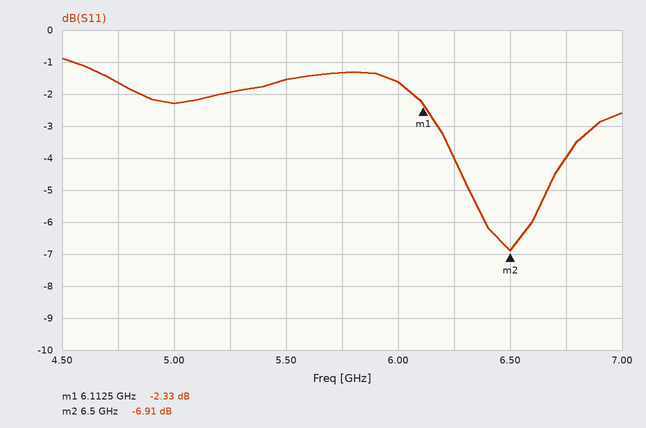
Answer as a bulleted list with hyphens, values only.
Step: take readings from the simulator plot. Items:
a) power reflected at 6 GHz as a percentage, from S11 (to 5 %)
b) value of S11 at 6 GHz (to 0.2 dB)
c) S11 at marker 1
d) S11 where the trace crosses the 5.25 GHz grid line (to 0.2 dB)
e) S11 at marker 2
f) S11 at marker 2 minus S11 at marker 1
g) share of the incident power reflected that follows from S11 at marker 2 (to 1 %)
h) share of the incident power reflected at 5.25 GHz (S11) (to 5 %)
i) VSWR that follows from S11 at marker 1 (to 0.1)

- 70 %
- -1.6 dB
- -2.33 dB
- -2.0 dB
- -6.91 dB
- -4.58 dB
- 20 %
- 65 %
- 7.5
